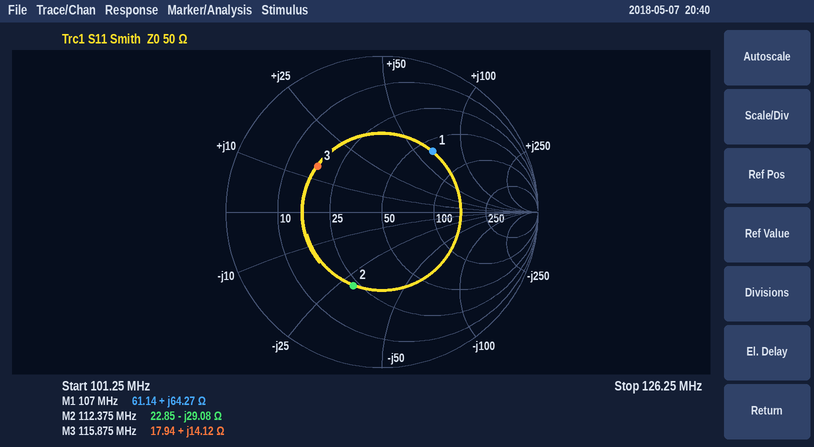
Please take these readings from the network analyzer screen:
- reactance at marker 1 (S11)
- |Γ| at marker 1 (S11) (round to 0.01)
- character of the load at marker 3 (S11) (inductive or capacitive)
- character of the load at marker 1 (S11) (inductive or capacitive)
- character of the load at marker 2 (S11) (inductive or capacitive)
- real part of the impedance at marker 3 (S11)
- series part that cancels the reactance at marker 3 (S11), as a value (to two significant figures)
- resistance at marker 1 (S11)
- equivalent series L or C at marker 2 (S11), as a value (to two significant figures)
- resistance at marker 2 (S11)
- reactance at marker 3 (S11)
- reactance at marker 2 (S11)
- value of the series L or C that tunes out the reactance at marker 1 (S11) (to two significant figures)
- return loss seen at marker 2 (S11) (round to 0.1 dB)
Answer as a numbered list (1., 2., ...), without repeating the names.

1. +64.27 Ω
2. 0.51
3. inductive
4. inductive
5. capacitive
6. 17.94 Ω
7. 97 pF
8. 61.14 Ω
9. 49 pF
10. 22.85 Ω
11. +14.12 Ω
12. -29.08 Ω
13. 23 pF
14. 5.9 dB
